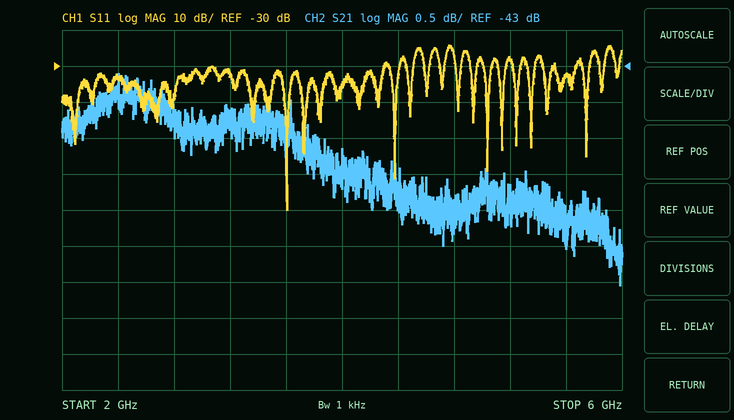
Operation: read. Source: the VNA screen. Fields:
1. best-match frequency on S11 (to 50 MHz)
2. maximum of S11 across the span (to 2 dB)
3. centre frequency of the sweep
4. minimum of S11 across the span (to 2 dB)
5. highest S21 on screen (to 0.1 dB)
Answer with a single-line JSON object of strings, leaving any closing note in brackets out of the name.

{"best-match frequency on S11": "3.60 GHz", "maximum of S11 across the span": "-24 dB", "centre frequency of the sweep": "4 GHz", "minimum of S11 across the span": "-70 dB", "highest S21 on screen": "-43.1 dB"}
